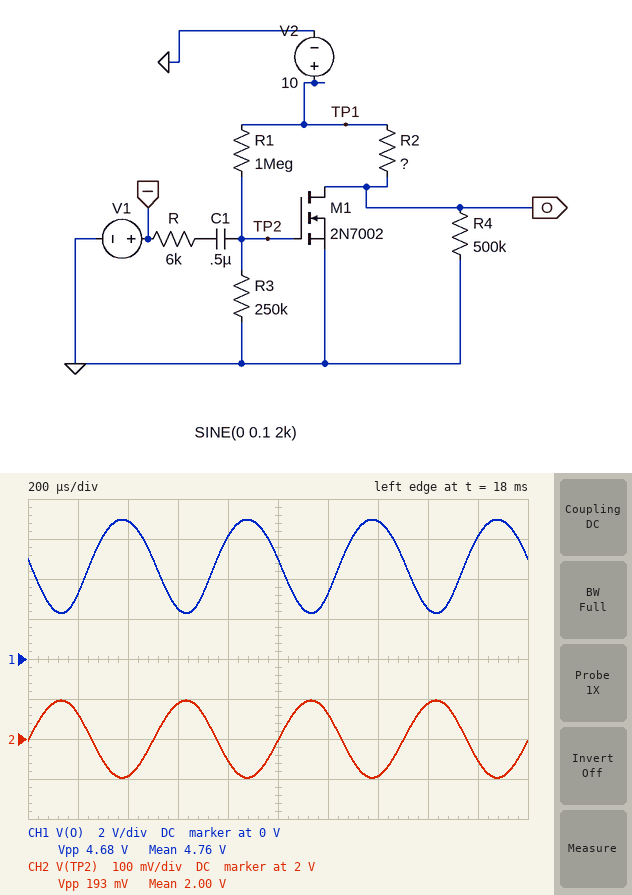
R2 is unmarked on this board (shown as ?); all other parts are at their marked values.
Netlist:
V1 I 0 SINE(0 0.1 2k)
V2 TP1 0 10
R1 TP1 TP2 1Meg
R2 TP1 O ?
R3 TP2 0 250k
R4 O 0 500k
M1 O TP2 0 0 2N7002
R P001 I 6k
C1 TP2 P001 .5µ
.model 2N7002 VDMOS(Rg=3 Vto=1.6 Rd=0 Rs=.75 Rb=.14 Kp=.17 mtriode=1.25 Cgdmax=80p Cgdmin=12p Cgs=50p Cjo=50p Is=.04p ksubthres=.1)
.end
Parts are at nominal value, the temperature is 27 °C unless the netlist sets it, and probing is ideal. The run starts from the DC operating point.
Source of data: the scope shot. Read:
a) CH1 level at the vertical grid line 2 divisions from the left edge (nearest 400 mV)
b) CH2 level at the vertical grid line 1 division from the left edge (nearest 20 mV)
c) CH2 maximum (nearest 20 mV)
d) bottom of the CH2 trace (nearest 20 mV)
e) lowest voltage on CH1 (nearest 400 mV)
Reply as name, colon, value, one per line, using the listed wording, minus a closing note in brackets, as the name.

CH1 level at the vertical grid line 2 divisions from the left edge: 6.8 V
CH2 level at the vertical grid line 1 division from the left edge: 2.06 V
CH2 maximum: 2.10 V
bottom of the CH2 trace: 1.90 V
lowest voltage on CH1: 2.4 V
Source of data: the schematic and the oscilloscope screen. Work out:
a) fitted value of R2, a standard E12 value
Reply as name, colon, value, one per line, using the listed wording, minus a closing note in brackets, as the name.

fitted value of R2, a standard E12 value: 390 Ω
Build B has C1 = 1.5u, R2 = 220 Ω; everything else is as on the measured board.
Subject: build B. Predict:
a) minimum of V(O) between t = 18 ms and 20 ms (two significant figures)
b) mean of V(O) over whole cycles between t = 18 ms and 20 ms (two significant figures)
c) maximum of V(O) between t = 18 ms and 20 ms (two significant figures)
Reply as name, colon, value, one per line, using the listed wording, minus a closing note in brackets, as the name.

minimum of V(O) between t = 18 ms and 20 ms: 5.6 V
mean of V(O) over whole cycles between t = 18 ms and 20 ms: 7.0 V
maximum of V(O) between t = 18 ms and 20 ms: 8.3 V
